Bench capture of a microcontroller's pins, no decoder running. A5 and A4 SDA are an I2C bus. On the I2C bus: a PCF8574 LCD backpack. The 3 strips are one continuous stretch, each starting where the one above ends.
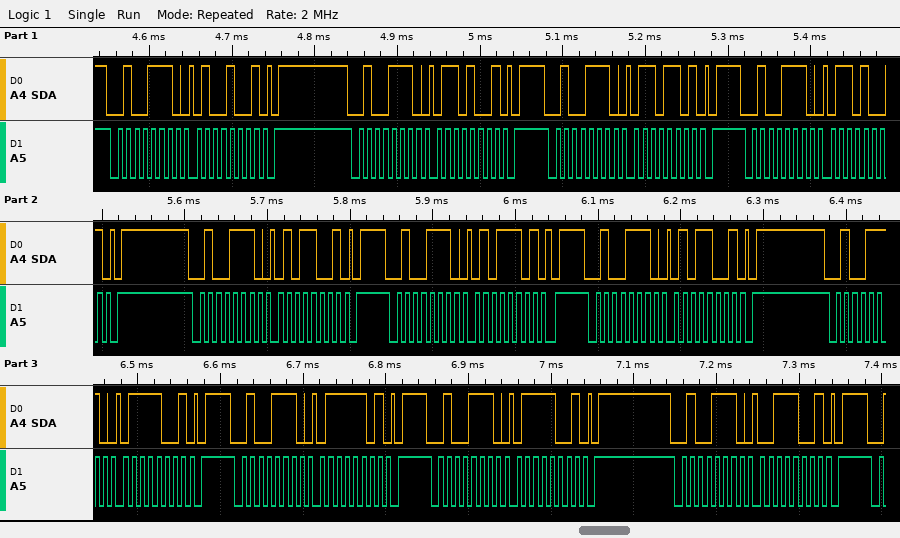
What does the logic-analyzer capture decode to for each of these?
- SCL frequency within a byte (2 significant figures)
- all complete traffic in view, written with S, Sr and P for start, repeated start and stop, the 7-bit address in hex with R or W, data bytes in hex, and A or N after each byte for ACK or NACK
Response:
100 kHz
S 27W A 49 A P S 27W A 69 A P S 27W A 6D A P S 27W A 69 A P S 27W A 59 A P S 27W A 5D A P S 27W A 59 A P S 27W A 79 A P S 27W A 7D A P S 27W A 79 A P S 27W A 39 A P
